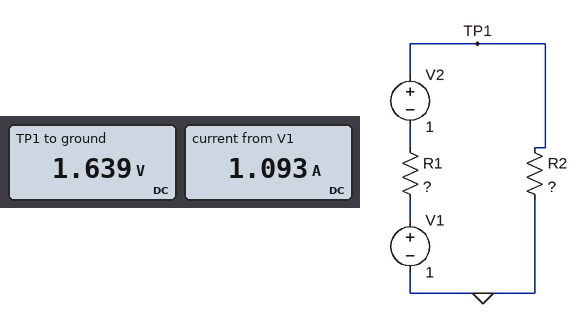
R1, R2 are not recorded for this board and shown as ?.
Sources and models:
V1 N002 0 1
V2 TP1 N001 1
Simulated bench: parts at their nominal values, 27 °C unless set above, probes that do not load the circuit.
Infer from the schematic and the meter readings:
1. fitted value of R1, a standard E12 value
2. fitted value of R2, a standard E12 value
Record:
0.33 Ω
1.5 Ω
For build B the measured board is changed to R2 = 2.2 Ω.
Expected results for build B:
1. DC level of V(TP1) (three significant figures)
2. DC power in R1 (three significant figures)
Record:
1.74 V
206 mW
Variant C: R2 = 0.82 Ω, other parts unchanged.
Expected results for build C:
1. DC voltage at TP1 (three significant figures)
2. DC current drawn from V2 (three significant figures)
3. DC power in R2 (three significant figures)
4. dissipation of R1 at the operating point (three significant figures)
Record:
1.43 V
1.74 A
2.48 W
998 mW
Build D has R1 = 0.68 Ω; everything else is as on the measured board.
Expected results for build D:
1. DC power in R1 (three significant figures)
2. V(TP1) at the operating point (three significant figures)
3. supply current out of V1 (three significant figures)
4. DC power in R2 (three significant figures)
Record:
572 mW
1.38 V
917 mA
1.26 W
